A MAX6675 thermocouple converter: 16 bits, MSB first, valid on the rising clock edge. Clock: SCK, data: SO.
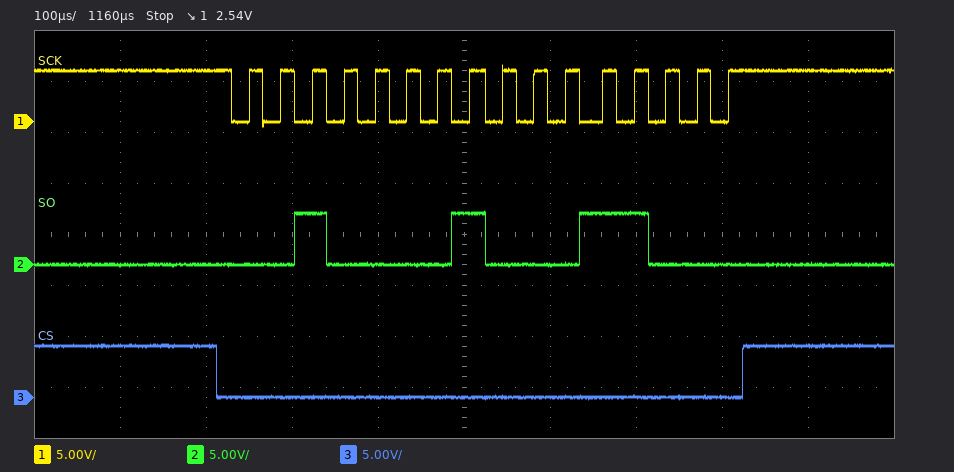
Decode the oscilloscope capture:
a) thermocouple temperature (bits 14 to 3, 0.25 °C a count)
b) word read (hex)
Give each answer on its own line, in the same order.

264.75 °C
0x2118
